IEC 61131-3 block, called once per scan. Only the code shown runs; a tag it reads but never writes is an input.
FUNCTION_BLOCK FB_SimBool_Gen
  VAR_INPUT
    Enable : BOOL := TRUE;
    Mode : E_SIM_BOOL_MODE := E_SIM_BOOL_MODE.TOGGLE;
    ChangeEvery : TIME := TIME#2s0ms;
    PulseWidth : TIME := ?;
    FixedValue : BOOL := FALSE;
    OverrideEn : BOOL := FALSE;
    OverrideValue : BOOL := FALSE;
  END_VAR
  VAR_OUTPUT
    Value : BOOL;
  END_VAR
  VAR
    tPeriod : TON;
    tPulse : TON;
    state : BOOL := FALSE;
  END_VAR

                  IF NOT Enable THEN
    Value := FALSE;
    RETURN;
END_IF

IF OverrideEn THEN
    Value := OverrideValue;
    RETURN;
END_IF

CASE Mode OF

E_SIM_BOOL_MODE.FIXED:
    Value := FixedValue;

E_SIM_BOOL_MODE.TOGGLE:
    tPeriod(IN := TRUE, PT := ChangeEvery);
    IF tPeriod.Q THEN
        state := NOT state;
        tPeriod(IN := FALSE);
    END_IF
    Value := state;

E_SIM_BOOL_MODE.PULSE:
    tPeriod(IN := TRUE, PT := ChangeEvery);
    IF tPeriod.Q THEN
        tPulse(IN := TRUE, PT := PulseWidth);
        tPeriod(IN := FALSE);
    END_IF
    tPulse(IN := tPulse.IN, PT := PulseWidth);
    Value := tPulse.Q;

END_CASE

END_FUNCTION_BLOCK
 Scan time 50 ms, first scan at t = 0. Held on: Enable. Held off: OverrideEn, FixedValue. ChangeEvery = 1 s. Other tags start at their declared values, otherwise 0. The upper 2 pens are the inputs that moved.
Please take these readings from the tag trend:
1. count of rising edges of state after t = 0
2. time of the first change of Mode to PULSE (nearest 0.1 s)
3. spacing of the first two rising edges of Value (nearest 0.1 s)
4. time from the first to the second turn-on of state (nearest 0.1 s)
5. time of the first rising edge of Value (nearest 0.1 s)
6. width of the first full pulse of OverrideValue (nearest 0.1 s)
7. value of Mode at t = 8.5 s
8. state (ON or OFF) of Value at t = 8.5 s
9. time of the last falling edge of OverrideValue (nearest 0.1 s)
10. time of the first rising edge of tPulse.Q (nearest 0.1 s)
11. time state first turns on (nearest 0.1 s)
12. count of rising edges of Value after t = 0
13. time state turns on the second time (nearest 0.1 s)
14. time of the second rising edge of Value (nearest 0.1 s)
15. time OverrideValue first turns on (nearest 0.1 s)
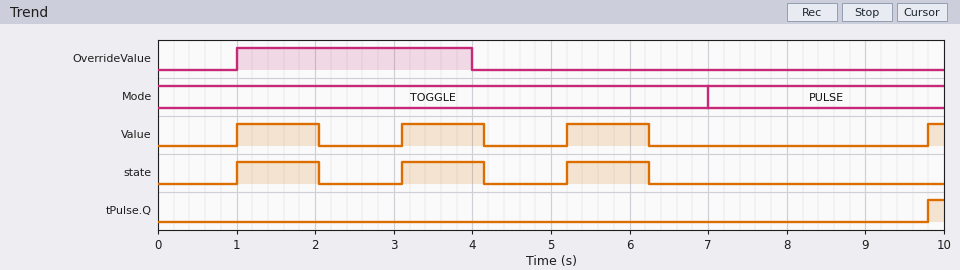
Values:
3
7.0 s
2.1 s
2.1 s
1.0 s
3.0 s
PULSE
OFF
4.0 s
9.8 s
1.0 s
4
3.1 s
3.1 s
1.0 s
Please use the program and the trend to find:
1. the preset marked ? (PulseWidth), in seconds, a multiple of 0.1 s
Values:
2.5 s
